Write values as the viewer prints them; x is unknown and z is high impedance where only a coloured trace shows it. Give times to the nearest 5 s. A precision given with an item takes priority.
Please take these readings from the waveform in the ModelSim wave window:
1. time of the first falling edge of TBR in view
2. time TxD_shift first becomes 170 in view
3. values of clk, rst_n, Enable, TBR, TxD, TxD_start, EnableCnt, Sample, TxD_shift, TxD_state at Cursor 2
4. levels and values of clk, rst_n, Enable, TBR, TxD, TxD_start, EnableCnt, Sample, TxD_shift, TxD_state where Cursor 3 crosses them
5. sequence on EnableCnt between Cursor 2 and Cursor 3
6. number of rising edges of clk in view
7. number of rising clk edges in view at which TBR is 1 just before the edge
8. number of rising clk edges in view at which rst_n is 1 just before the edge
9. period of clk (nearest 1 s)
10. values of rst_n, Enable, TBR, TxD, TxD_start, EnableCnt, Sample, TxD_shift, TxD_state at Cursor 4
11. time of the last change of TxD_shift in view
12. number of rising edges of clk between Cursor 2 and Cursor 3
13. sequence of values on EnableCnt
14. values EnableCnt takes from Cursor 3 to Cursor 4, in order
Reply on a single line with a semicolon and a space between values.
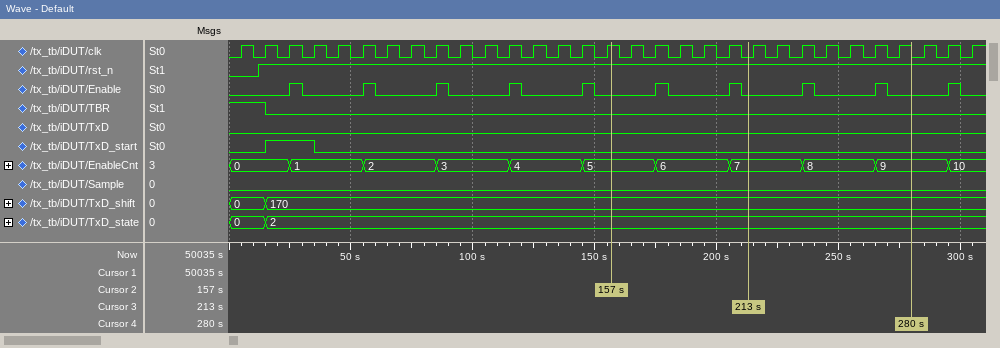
15 s; 15 s; clk=1, rst_n=1, Enable=0, TBR=0, TxD=0, TxD_start=0, EnableCnt=5, Sample=0, TxD_shift=170, TxD_state=2; clk=0, rst_n=1, Enable=0, TBR=0, TxD=0, TxD_start=0, EnableCnt=7, Sample=0, TxD_shift=170, TxD_state=2; 5, 6, 7; 31; 2; 30; 10 s; rst_n=1, Enable=0, TBR=0, TxD=0, TxD_start=0, EnableCnt=9, Sample=0, TxD_shift=170, TxD_state=2; 15 s; 5; 0, 1, 2, 3, 4, 5, 6, 7, 8, 9, 10; 7, 8, 9
